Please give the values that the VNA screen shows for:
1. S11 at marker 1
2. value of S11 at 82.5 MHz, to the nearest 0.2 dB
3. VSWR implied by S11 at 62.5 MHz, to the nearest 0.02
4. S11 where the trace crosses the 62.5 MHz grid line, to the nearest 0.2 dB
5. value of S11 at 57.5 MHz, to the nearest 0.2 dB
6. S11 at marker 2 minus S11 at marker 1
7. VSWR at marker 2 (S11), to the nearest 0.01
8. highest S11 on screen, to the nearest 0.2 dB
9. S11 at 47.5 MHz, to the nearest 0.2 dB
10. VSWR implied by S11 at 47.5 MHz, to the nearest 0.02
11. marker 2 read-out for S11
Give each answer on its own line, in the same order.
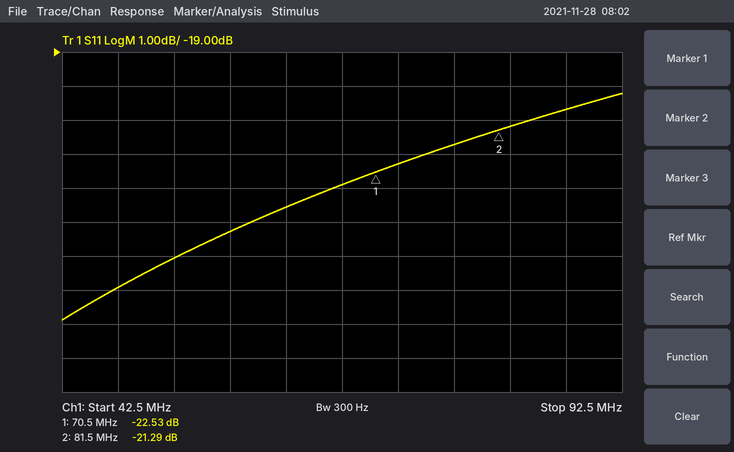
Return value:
-22.53 dB
-21.2 dB
1.14
-23.6 dB
-24.2 dB
1.24 dB
1.19
-20.2 dB
-26.0 dB
1.10
-21.29 dB
